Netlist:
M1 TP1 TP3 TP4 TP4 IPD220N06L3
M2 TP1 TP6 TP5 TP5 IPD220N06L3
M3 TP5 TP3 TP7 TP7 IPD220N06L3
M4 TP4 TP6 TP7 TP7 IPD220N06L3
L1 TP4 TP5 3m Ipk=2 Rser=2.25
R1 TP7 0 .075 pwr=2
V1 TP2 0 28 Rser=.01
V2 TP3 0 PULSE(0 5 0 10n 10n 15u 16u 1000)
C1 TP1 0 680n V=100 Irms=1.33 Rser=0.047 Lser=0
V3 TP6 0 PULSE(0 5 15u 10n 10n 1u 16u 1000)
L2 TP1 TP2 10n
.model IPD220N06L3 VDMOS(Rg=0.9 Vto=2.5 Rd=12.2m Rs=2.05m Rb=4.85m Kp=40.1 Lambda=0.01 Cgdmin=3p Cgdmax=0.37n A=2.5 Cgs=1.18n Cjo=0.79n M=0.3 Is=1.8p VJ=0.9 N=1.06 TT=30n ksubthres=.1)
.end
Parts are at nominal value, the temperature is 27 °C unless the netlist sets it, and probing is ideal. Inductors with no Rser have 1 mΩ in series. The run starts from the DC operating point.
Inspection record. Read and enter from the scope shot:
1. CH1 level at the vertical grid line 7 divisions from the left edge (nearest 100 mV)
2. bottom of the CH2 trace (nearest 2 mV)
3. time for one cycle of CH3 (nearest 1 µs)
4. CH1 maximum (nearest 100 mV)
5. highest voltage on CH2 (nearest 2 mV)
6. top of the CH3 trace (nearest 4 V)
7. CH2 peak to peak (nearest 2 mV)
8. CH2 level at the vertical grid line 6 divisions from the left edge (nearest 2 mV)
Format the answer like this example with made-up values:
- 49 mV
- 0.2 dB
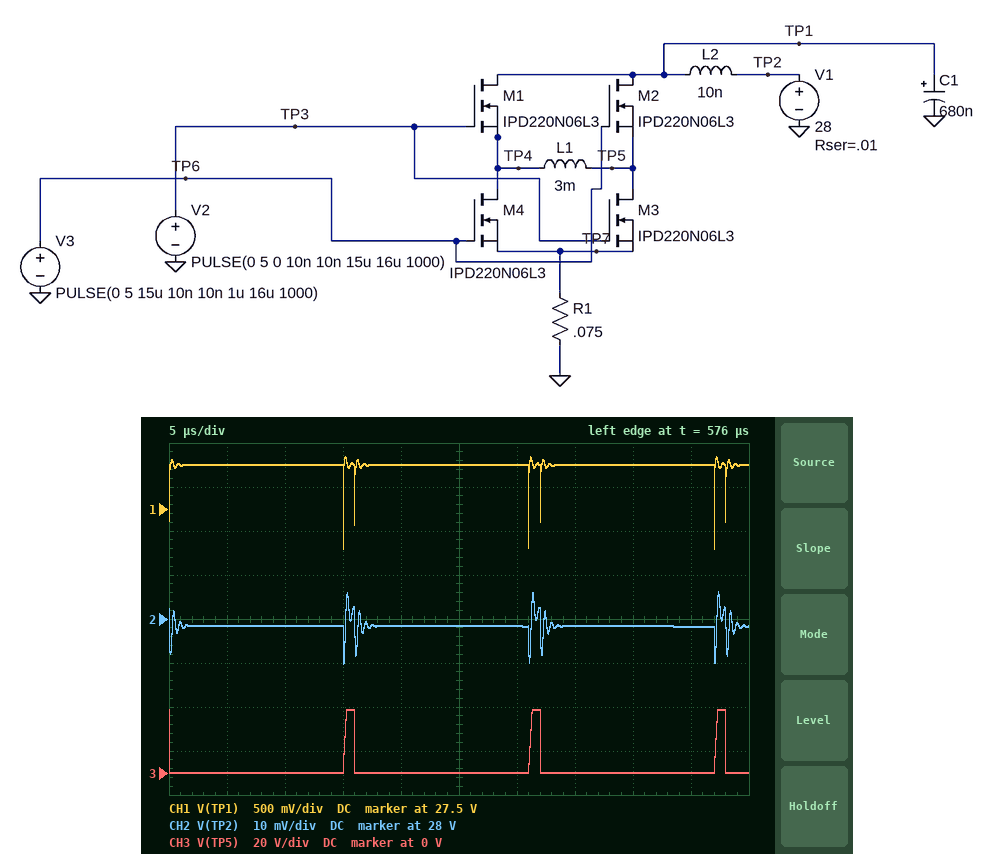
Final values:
- 28.0 V
- 27.990 V
- 16 µs
- 28.1 V
- 28.006 V
- 28 V
- 16 mV
- 27.998 V
